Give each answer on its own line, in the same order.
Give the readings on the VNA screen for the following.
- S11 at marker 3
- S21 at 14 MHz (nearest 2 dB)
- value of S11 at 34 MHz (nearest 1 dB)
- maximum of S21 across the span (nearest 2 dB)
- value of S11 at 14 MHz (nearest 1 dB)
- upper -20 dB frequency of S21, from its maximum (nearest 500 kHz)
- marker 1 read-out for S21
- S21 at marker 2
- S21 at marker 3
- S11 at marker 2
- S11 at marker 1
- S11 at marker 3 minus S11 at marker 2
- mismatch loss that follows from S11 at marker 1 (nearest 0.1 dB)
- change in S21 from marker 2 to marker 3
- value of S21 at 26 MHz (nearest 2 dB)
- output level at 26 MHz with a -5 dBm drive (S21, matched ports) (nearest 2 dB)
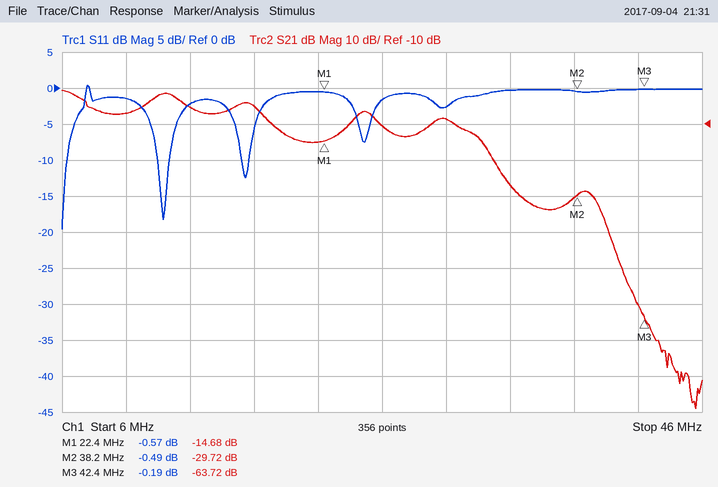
-0.19 dB
-6 dB
0 dB
0 dB
-2 dB
33.0 MHz
-14.68 dB
-29.72 dB
-63.72 dB
-0.49 dB
-0.57 dB
0.30 dB
9.1 dB
-34.00 dB
-10 dB
-16 dBm
